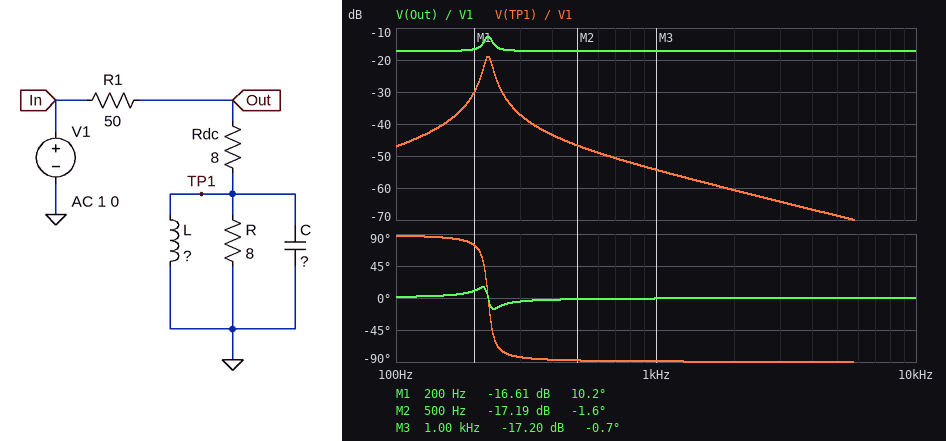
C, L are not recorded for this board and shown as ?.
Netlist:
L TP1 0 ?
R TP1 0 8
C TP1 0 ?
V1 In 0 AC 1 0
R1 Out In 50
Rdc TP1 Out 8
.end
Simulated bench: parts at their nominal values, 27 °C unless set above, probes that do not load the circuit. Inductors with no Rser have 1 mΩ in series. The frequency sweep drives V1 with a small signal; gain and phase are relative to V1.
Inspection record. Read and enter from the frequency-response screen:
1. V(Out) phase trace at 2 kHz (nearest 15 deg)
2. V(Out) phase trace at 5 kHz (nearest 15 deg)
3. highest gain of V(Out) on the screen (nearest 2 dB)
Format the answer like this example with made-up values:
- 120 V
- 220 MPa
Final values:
- 0 deg
- 0 deg
- -12 dB
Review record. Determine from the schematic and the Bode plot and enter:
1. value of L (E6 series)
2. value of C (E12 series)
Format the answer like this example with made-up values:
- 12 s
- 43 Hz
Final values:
- 330 µH
- 1.5 mF
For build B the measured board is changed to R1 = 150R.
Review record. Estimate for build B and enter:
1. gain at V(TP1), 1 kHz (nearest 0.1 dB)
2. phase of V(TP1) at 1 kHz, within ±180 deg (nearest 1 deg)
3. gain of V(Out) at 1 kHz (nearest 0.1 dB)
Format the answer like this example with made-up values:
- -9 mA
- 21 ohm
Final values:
- -63.0 dB
- -89 deg
- -25.9 dB
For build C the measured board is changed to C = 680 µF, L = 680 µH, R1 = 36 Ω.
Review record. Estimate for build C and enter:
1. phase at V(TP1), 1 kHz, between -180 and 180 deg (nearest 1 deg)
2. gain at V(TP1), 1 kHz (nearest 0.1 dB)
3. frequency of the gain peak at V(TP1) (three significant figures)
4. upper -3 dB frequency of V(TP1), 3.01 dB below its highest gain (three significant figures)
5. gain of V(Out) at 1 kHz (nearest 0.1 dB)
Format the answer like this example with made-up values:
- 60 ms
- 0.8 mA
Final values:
- -88 deg
- -45.0 dB
- 234 Hz
- 252 Hz
- -14.8 dB
